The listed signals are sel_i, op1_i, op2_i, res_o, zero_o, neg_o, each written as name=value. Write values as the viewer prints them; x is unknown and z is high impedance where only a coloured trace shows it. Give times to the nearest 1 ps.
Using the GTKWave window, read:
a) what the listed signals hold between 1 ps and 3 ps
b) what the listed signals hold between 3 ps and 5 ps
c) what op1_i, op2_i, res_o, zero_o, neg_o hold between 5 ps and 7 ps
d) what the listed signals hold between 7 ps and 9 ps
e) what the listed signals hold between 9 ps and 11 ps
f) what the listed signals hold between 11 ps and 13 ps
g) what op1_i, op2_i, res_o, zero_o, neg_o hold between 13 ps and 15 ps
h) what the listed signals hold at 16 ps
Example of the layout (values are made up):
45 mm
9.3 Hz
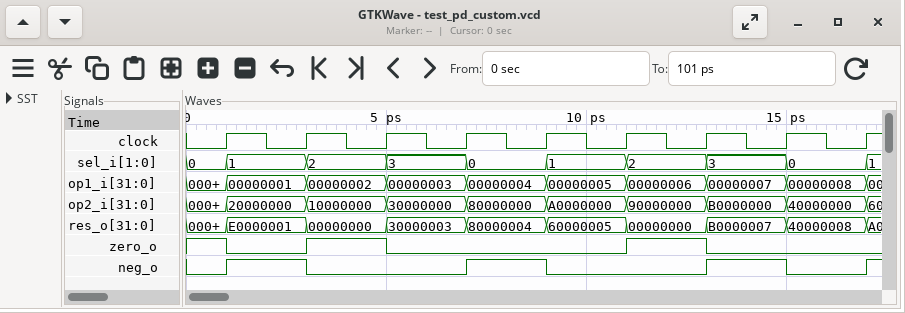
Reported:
sel_i=1, op1_i=00000001, op2_i=20000000, res_o=E0000001, zero_o=0, neg_o=1
sel_i=2, op1_i=00000002, op2_i=10000000, res_o=00000000, zero_o=1, neg_o=0
op1_i=00000003, op2_i=30000000, res_o=30000003, zero_o=0, neg_o=0
sel_i=0, op1_i=00000004, op2_i=80000000, res_o=80000004, zero_o=0, neg_o=1
sel_i=1, op1_i=00000005, op2_i=A0000000, res_o=60000005, zero_o=0, neg_o=0
sel_i=2, op1_i=00000006, op2_i=90000000, res_o=00000000, zero_o=1, neg_o=0
op1_i=00000007, op2_i=B0000000, res_o=B0000007, zero_o=0, neg_o=1
sel_i=0, op1_i=00000008, op2_i=40000000, res_o=40000008, zero_o=0, neg_o=0
